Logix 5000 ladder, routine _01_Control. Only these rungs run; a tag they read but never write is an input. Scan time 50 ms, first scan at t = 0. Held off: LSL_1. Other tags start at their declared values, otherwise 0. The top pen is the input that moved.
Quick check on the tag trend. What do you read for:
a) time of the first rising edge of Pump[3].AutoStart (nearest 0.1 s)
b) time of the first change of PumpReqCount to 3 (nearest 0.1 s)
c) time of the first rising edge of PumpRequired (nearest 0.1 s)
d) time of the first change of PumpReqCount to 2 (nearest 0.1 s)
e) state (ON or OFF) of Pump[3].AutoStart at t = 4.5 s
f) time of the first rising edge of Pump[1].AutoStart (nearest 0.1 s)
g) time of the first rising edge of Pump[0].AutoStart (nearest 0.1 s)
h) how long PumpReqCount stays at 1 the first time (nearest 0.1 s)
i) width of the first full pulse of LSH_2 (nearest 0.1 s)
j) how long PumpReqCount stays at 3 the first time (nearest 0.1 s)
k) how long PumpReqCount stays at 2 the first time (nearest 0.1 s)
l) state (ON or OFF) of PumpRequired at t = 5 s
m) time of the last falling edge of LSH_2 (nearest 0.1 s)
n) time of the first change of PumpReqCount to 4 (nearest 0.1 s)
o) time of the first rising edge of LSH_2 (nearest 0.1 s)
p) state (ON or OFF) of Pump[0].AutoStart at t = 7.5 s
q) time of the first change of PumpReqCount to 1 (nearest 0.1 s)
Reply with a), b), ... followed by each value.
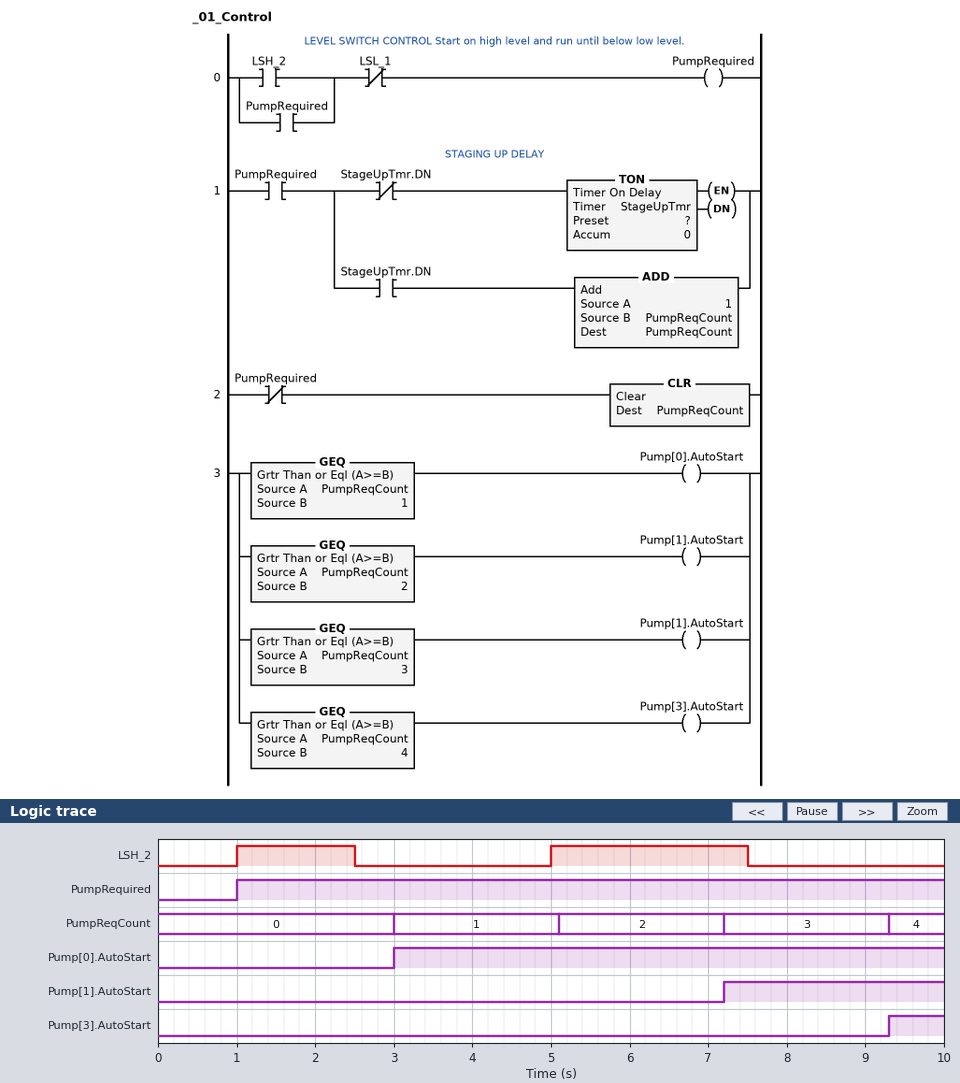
a) 9.3 s
b) 7.2 s
c) 1.0 s
d) 5.1 s
e) OFF
f) 7.2 s
g) 3.0 s
h) 2.1 s
i) 1.5 s
j) 2.1 s
k) 2.1 s
l) ON
m) 7.5 s
n) 9.3 s
o) 1.0 s
p) ON
q) 3.0 s
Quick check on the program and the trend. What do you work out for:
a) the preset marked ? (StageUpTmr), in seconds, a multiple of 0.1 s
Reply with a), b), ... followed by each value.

a) 2.0 s
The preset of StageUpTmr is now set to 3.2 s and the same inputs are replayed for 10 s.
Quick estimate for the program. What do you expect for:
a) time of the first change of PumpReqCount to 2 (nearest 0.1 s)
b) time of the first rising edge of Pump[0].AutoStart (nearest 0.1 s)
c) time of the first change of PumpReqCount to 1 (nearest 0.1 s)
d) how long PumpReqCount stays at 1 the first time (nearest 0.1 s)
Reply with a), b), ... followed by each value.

a) 7.5 s
b) 4.2 s
c) 4.2 s
d) 3.3 s
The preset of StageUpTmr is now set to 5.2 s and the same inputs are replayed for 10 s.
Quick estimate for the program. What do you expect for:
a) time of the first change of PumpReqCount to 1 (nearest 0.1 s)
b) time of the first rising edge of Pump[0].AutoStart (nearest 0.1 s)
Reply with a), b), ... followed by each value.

a) 6.2 s
b) 6.2 s
